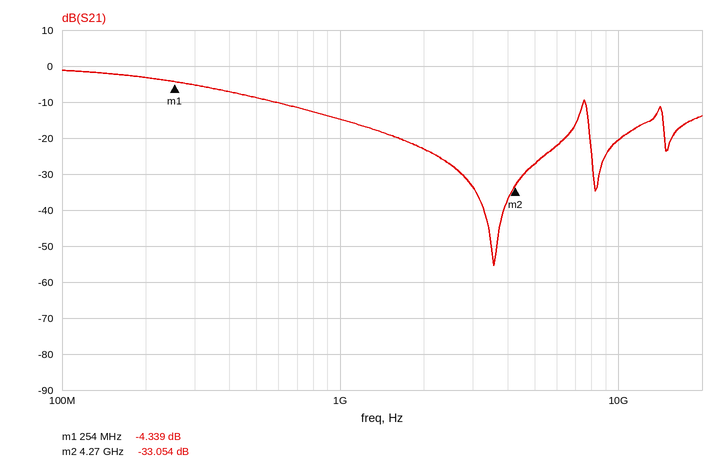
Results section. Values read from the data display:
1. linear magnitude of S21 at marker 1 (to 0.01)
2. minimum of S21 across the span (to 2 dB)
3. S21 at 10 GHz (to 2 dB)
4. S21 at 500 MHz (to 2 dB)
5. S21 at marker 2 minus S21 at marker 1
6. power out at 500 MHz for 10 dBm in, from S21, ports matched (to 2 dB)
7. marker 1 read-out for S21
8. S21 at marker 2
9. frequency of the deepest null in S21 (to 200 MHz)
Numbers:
0.61
-56 dB
-20 dB
-8 dB
-28.715 dB
2 dBm
-4.339 dB
-33.054 dB
3.6 GHz
